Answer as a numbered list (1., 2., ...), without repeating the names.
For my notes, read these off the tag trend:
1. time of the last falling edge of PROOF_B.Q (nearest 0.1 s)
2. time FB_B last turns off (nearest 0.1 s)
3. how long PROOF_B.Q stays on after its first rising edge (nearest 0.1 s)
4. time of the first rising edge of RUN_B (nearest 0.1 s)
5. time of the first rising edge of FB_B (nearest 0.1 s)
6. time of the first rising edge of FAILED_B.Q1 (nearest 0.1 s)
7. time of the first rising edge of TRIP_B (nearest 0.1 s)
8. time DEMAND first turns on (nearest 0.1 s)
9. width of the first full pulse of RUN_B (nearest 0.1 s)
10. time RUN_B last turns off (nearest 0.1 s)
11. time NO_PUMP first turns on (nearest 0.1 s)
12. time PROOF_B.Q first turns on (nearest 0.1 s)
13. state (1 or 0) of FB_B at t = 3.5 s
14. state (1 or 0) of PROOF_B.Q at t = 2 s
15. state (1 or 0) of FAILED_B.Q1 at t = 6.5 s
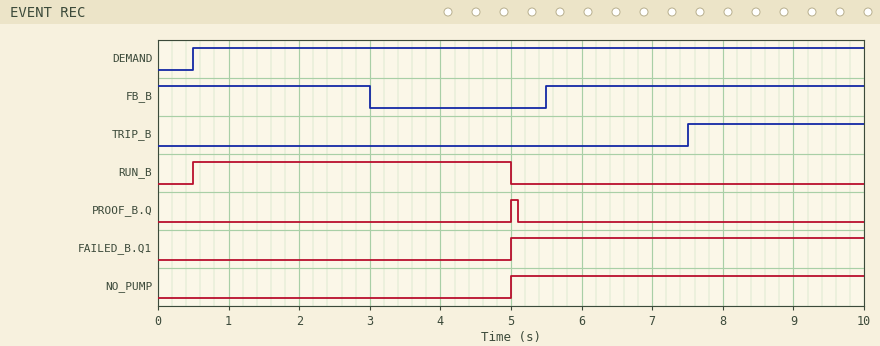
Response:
1. 5.1 s
2. 3.0 s
3. 0.1 s
4. 0.5 s
5. 5.5 s
6. 5.0 s
7. 7.5 s
8. 0.5 s
9. 4.5 s
10. 5.0 s
11. 5.0 s
12. 5.0 s
13. 0
14. 0
15. 1
